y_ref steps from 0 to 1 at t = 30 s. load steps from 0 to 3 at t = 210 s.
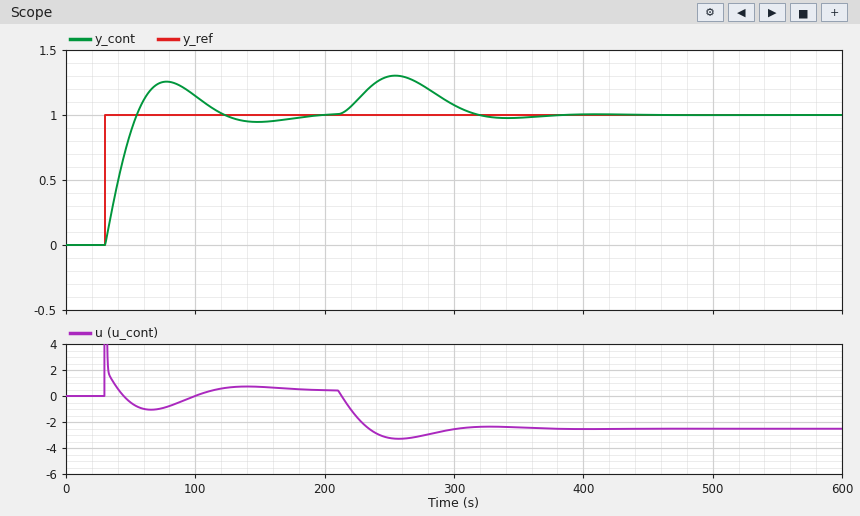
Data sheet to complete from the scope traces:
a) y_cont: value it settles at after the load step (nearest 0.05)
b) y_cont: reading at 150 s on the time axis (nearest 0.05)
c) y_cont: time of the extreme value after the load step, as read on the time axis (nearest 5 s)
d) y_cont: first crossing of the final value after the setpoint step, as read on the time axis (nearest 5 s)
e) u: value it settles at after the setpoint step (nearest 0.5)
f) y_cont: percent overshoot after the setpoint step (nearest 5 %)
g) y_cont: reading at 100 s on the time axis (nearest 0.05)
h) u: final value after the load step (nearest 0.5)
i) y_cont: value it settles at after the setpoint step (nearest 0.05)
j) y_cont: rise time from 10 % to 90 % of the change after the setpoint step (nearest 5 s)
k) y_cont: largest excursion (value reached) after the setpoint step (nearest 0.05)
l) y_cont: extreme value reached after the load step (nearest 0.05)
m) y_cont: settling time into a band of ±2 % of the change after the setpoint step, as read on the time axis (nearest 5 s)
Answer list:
1.00
0.95
255 s
55 s
0.5
25 %
1.15
-2.5
1.00
20 s
1.25
1.30
180 s
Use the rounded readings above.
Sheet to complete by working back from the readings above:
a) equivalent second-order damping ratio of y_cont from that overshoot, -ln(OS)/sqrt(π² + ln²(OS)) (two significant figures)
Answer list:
0.40
